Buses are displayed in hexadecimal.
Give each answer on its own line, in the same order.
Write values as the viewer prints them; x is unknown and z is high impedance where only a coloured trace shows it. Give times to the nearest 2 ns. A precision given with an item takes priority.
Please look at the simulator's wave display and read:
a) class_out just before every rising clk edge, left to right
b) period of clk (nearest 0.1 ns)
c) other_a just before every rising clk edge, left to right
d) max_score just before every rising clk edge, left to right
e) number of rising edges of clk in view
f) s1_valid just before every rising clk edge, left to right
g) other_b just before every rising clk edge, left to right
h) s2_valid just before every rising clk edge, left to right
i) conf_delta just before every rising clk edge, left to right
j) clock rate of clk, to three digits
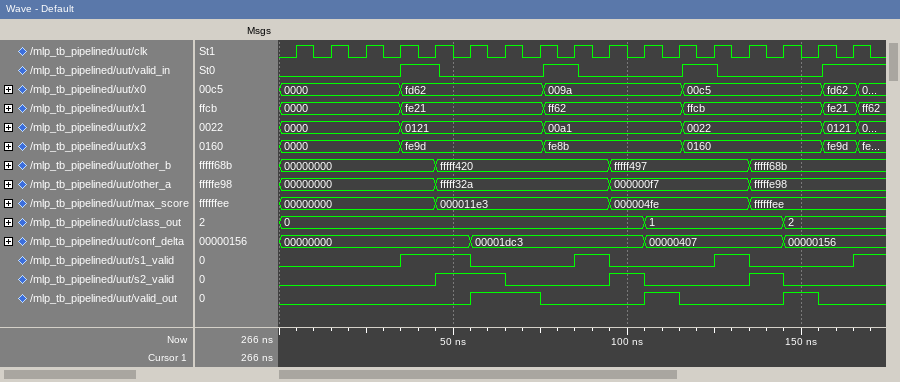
0, 0, 0, 0, 0, 0, 0, 0, 0, 0, 0, 1, 1, 1, 1, 2, 2
10 ns
00000000, 00000000, 00000000, 00000000, 00000000, fffff32a, fffff32a, fffff32a, fffff32a, fffff32a, 000000f7, 000000f7, 000000f7, 000000f7, fffffe98, fffffe98, fffffe98
00000000, 00000000, 00000000, 00000000, 00000000, 000011e3, 000011e3, 000011e3, 000011e3, 000011e3, 000004fe, 000004fe, 000004fe, 000004fe, ffffffee, ffffffee, ffffffee
17
0 0 0 0 1 1 0 0 0 1 0 0 0 1 0 0 0
00000000, 00000000, 00000000, 00000000, 00000000, fffff420, fffff420, fffff420, fffff420, fffff420, fffff497, fffff497, fffff497, fffff497, fffff68b, fffff68b, fffff68b
0 0 0 0 0 1 1 0 0 0 1 0 0 0 1 0 0
00000000, 00000000, 00000000, 00000000, 00000000, 00000000, 00001dc3, 00001dc3, 00001dc3, 00001dc3, 00001dc3, 00000407, 00000407, 00000407, 00000407, 00000156, 00000156
100 MHz
